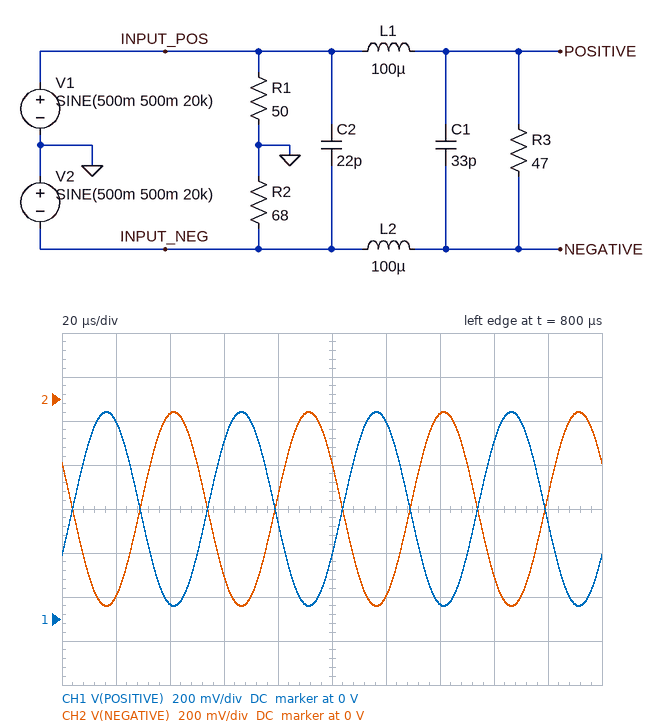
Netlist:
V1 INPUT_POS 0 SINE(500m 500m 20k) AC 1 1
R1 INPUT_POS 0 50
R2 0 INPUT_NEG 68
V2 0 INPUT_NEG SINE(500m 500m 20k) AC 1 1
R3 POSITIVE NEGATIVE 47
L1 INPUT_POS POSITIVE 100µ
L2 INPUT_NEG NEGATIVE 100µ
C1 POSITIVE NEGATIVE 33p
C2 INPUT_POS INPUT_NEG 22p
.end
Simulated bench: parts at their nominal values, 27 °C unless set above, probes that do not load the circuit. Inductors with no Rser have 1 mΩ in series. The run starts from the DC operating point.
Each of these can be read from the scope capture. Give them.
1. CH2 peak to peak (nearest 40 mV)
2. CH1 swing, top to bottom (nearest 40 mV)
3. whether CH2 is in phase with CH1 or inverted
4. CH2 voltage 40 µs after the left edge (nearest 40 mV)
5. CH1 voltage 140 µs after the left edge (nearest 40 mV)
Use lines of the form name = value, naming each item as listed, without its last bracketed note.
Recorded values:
CH2 peak to peak = 880 mV
CH1 swing, top to bottom = 880 mV
whether CH2 is in phase with CH1 or inverted = inverted
CH2 voltage 40 µs after the left edge = -80 mV
CH1 voltage 140 µs after the left edge = 80 mV
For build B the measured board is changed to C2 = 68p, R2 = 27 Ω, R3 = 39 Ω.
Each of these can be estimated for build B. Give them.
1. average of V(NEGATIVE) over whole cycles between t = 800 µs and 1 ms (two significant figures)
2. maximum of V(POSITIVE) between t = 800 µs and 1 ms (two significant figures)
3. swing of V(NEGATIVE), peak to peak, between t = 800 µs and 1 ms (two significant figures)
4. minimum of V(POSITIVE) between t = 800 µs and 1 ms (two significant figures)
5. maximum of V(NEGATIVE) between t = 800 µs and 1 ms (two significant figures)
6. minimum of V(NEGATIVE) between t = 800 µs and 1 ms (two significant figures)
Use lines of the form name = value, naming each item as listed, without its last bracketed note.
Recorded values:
average of V(NEGATIVE) over whole cycles between t = 800 µs and 1 ms = -500 mV
maximum of V(POSITIVE) between t = 800 µs and 1 ms = 920 mV
swing of V(NEGATIVE), peak to peak, between t = 800 µs and 1 ms = 840 mV
minimum of V(POSITIVE) between t = 800 µs and 1 ms = 80 mV
maximum of V(NEGATIVE) between t = 800 µs and 1 ms = -80 mV
minimum of V(NEGATIVE) between t = 800 µs and 1 ms = -920 mV
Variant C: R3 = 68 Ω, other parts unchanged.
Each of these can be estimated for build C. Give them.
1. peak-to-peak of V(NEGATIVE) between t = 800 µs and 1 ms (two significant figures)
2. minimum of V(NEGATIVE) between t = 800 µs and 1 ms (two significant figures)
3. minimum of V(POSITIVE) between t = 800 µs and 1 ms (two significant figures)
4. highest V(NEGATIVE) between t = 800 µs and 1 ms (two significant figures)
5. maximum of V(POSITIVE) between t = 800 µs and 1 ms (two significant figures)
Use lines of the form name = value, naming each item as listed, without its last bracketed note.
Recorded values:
peak-to-peak of V(NEGATIVE) between t = 800 µs and 1 ms = 940 mV
minimum of V(NEGATIVE) between t = 800 µs and 1 ms = -970 mV
minimum of V(POSITIVE) between t = 800 µs and 1 ms = 31 mV
highest V(NEGATIVE) between t = 800 µs and 1 ms = -31 mV
maximum of V(POSITIVE) between t = 800 µs and 1 ms = 970 mV
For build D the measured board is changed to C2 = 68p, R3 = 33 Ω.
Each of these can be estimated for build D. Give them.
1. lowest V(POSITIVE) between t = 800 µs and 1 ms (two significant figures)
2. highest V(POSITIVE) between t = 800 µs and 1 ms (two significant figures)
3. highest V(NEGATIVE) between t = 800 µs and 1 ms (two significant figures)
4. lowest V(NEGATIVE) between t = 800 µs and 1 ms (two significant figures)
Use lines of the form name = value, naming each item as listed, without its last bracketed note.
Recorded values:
lowest V(POSITIVE) between t = 800 µs and 1 ms = 100 mV
highest V(POSITIVE) between t = 800 µs and 1 ms = 900 mV
highest V(NEGATIVE) between t = 800 µs and 1 ms = -100 mV
lowest V(NEGATIVE) between t = 800 µs and 1 ms = -900 mV
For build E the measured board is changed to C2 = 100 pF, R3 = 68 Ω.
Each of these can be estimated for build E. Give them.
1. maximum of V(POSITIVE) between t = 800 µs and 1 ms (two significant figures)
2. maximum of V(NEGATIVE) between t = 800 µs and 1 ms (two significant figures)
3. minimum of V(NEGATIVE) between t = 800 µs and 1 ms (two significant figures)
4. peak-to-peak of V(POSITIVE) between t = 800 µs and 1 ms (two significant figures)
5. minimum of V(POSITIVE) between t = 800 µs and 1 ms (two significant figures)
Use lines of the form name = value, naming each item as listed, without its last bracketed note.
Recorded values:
maximum of V(POSITIVE) between t = 800 µs and 1 ms = 970 mV
maximum of V(NEGATIVE) between t = 800 µs and 1 ms = -31 mV
minimum of V(NEGATIVE) between t = 800 µs and 1 ms = -970 mV
peak-to-peak of V(POSITIVE) between t = 800 µs and 1 ms = 940 mV
minimum of V(POSITIVE) between t = 800 µs and 1 ms = 31 mV
